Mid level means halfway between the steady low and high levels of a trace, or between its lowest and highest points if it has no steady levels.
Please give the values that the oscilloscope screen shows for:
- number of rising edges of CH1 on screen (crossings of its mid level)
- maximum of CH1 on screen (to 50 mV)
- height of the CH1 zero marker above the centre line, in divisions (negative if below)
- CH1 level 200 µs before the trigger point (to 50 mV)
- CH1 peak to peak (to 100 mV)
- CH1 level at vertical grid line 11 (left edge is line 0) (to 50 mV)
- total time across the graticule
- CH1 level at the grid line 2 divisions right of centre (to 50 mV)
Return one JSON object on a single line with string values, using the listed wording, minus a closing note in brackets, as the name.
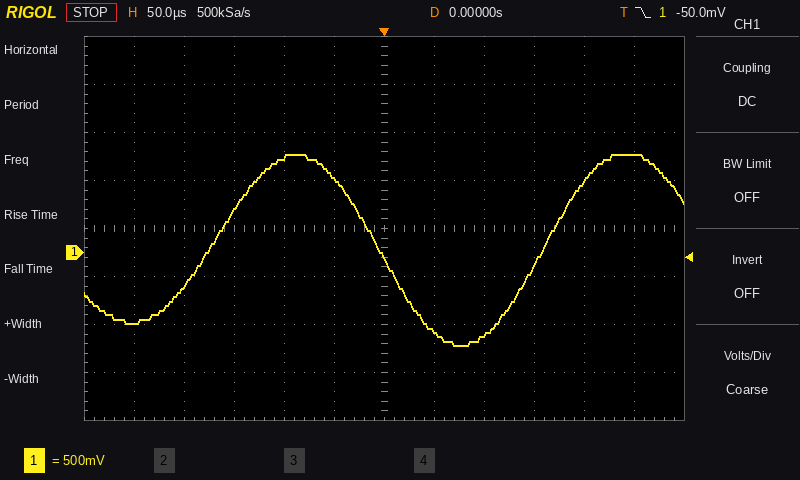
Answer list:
{"number of rising edges of CH1 on screen": "2", "maximum of CH1 on screen": "1.00 V", "height of the CH1 zero marker above the centre line, in divisions": "-0.5 div", "CH1 level 200 µs before the trigger point": "-350 mV", "CH1 peak to peak": "2.00 V", "CH1 level at vertical grid line 11 (left edge is line 0)": "1.00 V", "total time across the graticule": "600 µs", "CH1 level at the grid line 2 divisions right of centre": "-850 mV"}
